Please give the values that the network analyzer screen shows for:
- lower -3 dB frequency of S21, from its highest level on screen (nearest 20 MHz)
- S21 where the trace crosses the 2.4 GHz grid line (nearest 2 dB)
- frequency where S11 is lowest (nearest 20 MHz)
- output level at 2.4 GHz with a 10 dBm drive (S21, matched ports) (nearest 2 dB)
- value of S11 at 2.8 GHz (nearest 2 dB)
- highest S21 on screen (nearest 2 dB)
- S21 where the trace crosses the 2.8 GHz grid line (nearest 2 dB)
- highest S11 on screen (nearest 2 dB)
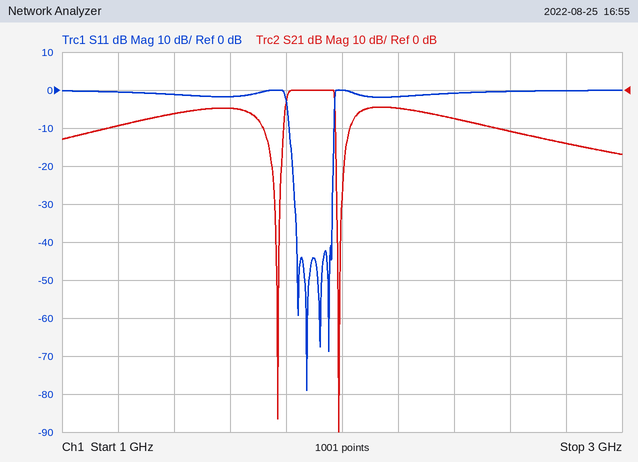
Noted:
1.80 GHz
-8 dB
1.88 GHz
2 dBm
0 dB
0 dB
-14 dB
0 dB
